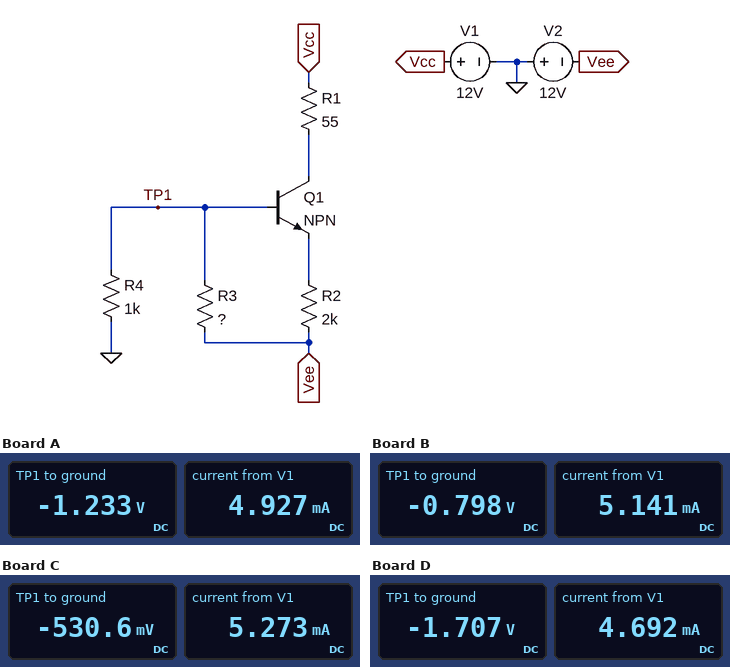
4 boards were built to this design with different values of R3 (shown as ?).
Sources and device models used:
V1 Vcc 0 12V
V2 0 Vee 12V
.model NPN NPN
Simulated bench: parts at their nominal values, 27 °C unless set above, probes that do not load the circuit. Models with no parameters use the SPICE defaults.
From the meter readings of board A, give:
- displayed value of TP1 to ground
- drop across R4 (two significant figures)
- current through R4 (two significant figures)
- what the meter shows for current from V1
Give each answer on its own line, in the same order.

-1.233 V
1.2 V
1.2 mA
4.927 mA
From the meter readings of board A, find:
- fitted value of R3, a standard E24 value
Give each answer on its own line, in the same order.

9.1 kΩ
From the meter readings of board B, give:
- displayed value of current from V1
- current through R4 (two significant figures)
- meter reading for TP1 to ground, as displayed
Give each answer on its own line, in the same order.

5.141 mA
800 µA
-0.798 V
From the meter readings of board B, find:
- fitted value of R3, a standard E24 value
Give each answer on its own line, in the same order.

15 kΩ
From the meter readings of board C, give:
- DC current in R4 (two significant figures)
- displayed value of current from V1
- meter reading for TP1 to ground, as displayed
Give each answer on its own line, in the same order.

530 µA
5.273 mA
-530.6 mV
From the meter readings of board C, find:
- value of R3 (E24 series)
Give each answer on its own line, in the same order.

24 kΩ
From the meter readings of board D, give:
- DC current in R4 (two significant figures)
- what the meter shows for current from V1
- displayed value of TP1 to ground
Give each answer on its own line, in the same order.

1.7 mA
4.692 mA
-1.707 V
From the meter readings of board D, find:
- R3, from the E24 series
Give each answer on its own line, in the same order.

6.2 kΩ
